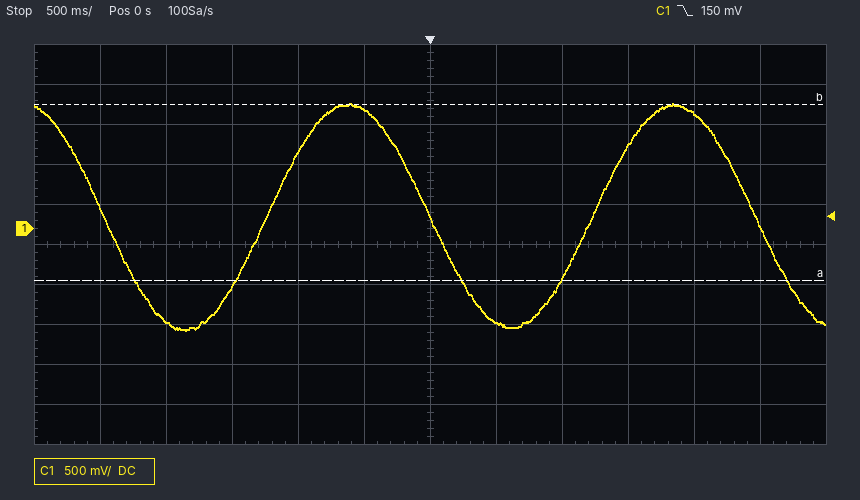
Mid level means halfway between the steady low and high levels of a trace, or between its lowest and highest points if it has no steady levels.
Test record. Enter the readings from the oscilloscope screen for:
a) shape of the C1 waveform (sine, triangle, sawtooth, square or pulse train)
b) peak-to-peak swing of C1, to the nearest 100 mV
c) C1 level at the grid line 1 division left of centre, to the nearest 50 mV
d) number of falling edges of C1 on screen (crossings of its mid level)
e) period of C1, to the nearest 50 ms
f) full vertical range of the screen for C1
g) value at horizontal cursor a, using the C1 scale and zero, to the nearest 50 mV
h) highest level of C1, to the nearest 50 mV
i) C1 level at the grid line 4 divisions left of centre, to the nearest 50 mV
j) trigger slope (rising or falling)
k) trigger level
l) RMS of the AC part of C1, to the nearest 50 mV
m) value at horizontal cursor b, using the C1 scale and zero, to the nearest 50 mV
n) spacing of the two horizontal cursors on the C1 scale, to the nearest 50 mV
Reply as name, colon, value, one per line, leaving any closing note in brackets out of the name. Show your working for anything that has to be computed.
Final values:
shape of the C1 waveform: sine
peak-to-peak swing of C1, to the nearest 100 mV: 2.80 V
C1 level at the grid line 1 division left of centre, to the nearest 50 mV: 1.50 V
number of falling edges of C1 on screen: 3
period of C1, to the nearest 50 ms: 2.45 s
full vertical range of the screen for C1: 5 V
value at horizontal cursor a, using the C1 scale and zero, to the nearest 50 mV: -650 mV
highest level of C1, to the nearest 50 mV: 1.55 V
C1 level at the grid line 4 divisions left of centre, to the nearest 50 mV: -1.15 V
trigger slope: falling
trigger level: 150 mV
RMS of the AC part of C1, to the nearest 50 mV: 2.80 V / (2√2) ≈ 0.990 V, so 1.00 V to the nearest 50 mV
value at horizontal cursor b, using the C1 scale and zero, to the nearest 50 mV: 1.55 V
spacing of the two horizontal cursors on the C1 scale, to the nearest 50 mV: 2.20 V
